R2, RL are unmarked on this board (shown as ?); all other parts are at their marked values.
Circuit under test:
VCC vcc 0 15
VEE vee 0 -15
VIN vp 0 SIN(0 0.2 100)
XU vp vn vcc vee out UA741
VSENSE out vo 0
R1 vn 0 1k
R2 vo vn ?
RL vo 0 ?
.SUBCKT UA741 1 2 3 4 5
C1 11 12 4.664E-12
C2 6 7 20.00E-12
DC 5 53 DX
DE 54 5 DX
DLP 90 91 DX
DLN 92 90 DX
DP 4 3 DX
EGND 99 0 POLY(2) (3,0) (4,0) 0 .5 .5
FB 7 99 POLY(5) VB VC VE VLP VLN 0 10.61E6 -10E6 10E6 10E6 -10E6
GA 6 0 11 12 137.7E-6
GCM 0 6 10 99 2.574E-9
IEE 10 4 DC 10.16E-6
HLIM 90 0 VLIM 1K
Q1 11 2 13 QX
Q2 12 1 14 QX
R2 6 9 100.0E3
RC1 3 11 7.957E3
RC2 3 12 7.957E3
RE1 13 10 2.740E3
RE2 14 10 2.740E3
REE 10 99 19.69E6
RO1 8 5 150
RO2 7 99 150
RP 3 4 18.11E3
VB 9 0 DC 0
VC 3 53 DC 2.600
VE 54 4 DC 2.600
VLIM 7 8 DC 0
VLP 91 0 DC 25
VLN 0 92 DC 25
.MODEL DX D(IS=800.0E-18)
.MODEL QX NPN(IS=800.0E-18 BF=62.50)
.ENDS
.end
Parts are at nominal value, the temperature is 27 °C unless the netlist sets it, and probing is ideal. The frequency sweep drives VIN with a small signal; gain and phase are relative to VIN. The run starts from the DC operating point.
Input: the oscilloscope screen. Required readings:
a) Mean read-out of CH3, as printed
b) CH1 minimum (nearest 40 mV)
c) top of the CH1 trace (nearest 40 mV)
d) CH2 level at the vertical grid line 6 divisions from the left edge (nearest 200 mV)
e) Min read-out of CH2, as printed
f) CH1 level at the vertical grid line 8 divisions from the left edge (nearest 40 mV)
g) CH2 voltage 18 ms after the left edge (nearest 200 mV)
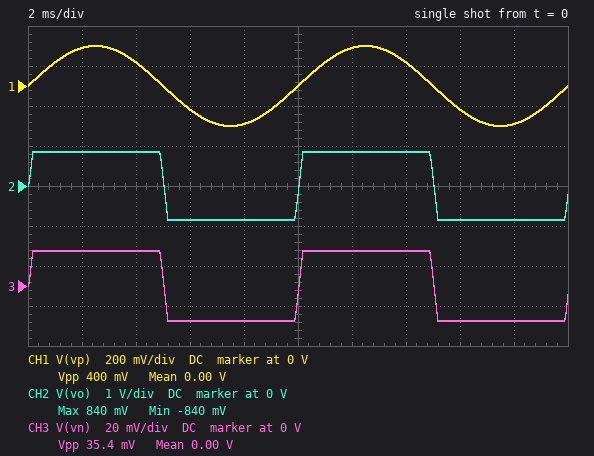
0.00 V
-200 mV
200 mV
800 mV
-840 mV
-120 mV
-800 mV
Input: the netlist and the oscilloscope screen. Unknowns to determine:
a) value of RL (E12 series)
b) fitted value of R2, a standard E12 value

33 Ω
47 kΩ
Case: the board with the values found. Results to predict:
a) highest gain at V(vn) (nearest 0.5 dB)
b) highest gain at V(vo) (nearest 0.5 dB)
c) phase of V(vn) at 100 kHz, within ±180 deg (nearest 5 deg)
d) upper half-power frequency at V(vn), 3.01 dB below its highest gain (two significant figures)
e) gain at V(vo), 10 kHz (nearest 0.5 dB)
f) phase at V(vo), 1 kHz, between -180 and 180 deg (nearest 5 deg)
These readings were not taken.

0 dB
33.5 dB
-90 deg
4.1 kHz
25.0 dB
-15 deg
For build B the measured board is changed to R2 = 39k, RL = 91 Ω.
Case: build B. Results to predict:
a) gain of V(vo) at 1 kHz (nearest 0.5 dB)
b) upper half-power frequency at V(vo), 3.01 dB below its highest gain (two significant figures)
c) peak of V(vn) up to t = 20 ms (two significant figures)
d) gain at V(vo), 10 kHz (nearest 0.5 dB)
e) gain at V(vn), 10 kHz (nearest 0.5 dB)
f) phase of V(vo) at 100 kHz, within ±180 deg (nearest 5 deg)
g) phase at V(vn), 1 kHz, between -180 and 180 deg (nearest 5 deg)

32.0 dB
10 kHz
58 mV
29.0 dB
-3.0 dB
-85 deg
-5 deg
